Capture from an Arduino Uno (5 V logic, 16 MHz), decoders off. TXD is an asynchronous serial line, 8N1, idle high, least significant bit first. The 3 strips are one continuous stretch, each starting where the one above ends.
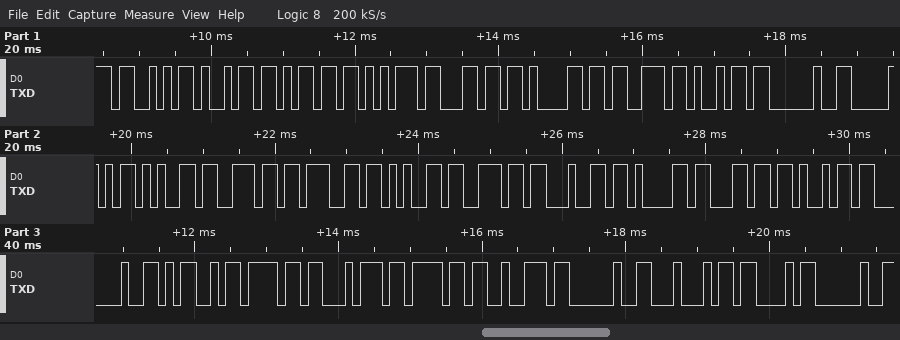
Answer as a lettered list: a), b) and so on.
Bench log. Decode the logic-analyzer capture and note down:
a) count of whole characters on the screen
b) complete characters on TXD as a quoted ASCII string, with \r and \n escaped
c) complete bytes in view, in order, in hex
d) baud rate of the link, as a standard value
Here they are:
a) 29
b) "Simulasi Pengendali Motor DC "
c) 0x53 0x69 0x6D 0x75 0x6C 0x61 0x73 0x69 0x20 0x50 0x65 0x6E 0x67 0x65 0x6E 0x64 0x61 0x6C 0x69 0x20 0x4D 0x6F 0x74 0x6F 0x72 0x20 0x44 0x43 0x20
d) 9600 baud
